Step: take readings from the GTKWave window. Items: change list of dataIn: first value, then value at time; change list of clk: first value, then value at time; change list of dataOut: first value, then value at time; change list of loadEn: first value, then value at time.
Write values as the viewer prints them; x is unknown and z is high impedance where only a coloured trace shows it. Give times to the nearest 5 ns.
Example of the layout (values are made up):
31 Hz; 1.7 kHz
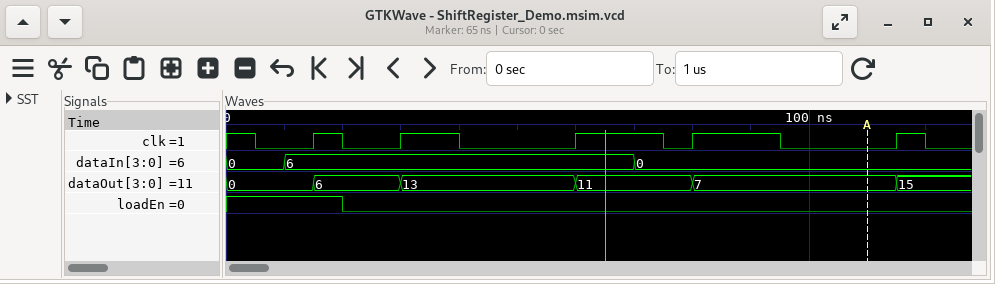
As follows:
0, 6 at 10 ns, 0 at 70 ns; 1, 0 at 5 ns, 1 at 15 ns, 0 at 20 ns, 1 at 30 ns, 0 at 40 ns, 1 at 60 ns, 0 at 75 ns, 1 at 80 ns, 0 at 95 ns, 1 at 115 ns, 0 at 120 ns; 0, 6 at 15 ns, 13 at 30 ns, 11 at 60 ns, 7 at 80 ns, 15 at 115 ns; 1, 0 at 20 ns
